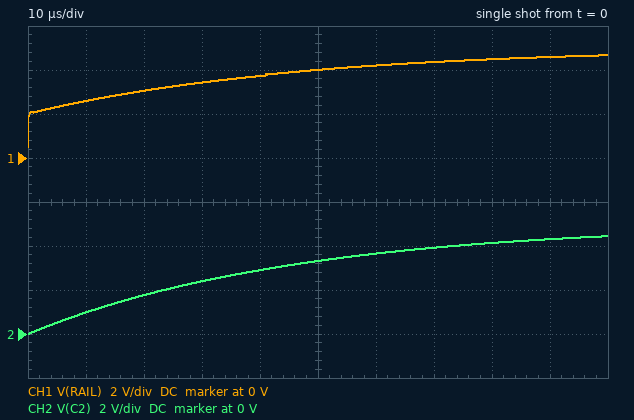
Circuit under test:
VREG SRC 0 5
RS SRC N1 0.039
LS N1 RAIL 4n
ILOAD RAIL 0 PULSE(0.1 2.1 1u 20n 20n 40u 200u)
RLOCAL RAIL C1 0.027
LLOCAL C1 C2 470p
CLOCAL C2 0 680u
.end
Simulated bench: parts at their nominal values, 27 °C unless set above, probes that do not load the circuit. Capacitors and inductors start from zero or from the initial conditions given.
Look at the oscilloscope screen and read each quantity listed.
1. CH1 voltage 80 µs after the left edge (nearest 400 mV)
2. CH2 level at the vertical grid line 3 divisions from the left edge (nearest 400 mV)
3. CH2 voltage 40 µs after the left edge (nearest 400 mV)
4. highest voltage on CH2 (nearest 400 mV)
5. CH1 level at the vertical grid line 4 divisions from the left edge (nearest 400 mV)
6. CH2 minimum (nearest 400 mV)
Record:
4.4 V
2.4 V
2.8 V
4.4 V
3.6 V
0 V
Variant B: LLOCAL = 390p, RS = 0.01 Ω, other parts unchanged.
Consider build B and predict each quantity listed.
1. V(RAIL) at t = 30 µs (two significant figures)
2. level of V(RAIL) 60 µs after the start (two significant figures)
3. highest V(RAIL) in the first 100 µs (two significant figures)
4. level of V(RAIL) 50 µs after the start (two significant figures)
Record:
4.6 V
4.9 V
5.0 V
4.8 V
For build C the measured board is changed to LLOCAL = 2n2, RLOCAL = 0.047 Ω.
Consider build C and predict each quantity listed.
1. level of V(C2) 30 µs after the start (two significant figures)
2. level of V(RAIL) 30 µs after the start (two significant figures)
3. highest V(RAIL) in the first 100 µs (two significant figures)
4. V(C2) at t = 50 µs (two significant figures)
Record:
2.0 V
3.6 V
4.6 V
2.8 V
